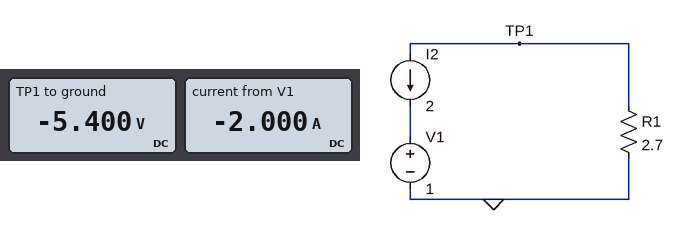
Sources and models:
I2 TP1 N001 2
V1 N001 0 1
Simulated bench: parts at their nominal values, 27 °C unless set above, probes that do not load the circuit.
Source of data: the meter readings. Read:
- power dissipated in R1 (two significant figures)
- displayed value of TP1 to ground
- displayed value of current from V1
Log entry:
11 W
-5.400 V
-2.000 A
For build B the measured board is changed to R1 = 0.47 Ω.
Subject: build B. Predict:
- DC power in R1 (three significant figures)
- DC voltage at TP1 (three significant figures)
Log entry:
1.88 W
-940 mV
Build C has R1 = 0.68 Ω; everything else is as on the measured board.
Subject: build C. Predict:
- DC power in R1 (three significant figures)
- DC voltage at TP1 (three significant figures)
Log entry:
2.72 W
-1.36 V
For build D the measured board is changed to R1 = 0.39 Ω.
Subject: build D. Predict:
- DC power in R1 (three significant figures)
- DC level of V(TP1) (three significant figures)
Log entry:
1.56 W
-780 mV
